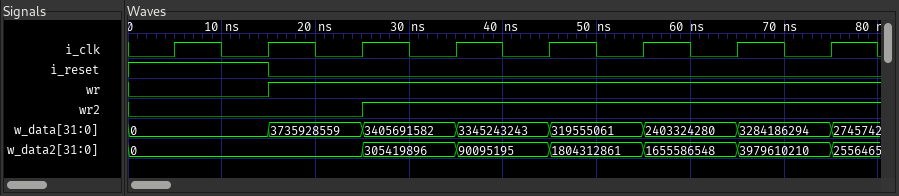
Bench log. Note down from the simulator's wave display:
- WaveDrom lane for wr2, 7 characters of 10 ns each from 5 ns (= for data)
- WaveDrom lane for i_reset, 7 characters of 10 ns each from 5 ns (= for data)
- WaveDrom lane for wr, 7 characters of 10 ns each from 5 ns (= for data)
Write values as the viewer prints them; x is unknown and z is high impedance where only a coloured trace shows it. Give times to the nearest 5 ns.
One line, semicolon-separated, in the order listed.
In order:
{name: 'wr2', wave: '0.1....'}; {name: 'i_reset', wave: '10.....'}; {name: 'wr', wave: '01.....'}
